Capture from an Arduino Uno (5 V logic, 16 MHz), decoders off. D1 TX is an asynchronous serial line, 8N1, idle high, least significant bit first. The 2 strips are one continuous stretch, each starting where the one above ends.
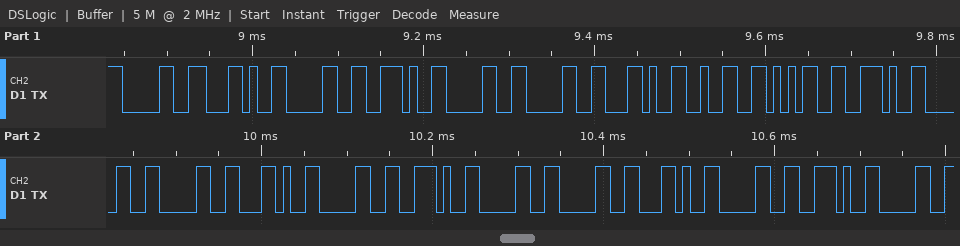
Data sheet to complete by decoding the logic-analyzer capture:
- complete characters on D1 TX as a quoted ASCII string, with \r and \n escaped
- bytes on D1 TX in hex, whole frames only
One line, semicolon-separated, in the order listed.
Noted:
"0,0.00,25.00,0.00,0.0"; 30 2C 30 2E 30 30 2C 32 35 2E 30 30 2C 30 2E 30 30 2C 30 2E 30
